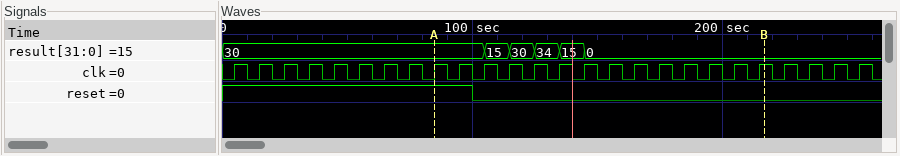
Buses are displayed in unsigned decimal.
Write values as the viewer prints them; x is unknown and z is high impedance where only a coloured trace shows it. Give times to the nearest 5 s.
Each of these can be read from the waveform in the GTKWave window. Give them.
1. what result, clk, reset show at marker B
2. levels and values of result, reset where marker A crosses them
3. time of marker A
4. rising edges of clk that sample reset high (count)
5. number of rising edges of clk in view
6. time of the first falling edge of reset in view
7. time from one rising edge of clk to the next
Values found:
result=0, clk=1, reset=0
result=30, reset=1
85 s
10
26
100 s
10 s
